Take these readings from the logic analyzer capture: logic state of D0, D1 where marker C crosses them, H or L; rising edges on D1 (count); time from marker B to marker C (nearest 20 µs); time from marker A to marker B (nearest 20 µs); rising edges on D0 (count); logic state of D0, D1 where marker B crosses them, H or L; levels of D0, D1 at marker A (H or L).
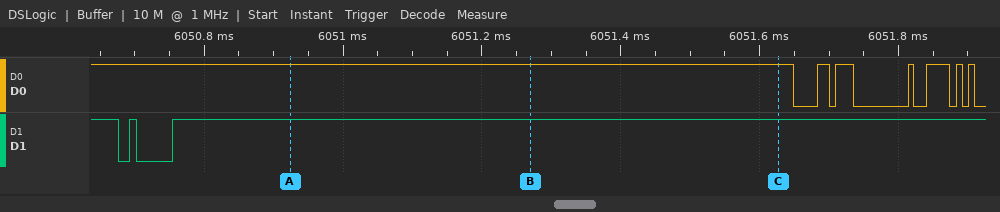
D0=H, D1=H
2
360 µs
340 µs
6
D0=H, D1=H
D0=H, D1=H
